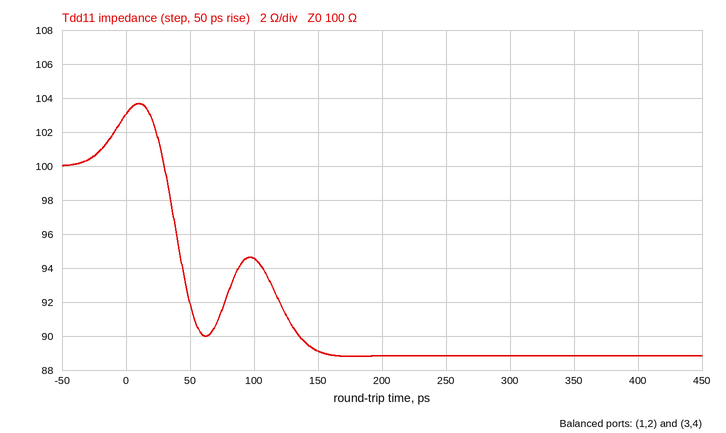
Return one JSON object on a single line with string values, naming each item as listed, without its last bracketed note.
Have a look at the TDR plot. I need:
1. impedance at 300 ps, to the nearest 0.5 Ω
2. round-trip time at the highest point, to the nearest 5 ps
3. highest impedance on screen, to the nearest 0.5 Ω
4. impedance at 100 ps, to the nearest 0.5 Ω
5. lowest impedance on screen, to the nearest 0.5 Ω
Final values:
{"impedance at 300 ps, to the nearest 0.5 Ω": "89.0 Ω", "round-trip time at the highest point, to the nearest 5 ps": "10 ps", "highest impedance on screen, to the nearest 0.5 Ω": "103.5 Ω", "impedance at 100 ps, to the nearest 0.5 Ω": "94.5 Ω", "lowest impedance on screen, to the nearest 0.5 Ω": "89.0 Ω"}
